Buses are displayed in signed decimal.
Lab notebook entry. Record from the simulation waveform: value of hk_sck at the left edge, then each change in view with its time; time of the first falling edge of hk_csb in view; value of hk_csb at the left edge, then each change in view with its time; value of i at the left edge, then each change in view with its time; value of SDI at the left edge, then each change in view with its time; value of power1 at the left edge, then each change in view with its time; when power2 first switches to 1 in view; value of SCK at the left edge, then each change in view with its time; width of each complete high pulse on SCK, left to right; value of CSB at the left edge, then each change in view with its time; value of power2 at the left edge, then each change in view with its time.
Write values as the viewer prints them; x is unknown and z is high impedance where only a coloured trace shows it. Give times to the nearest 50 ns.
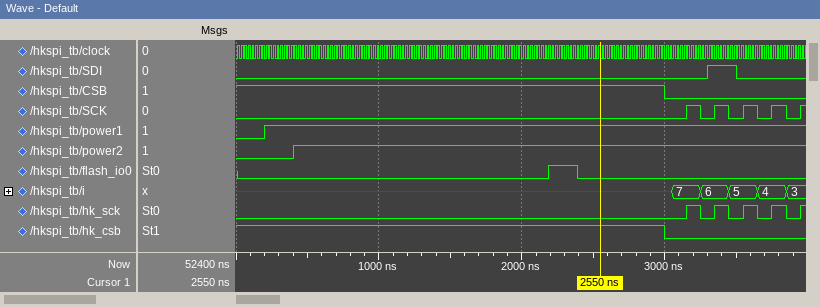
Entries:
0, 1 at 3150 ns, 0 at 3250 ns, 1 at 3350 ns, 0 at 3450 ns, 1 at 3550 ns, 0 at 3650 ns, 1 at 3750 ns, 0 at 3850 ns, 1 at 3950 ns
3000 ns
1, 0 at 3000 ns
x, 7 at 3050 ns, 6 at 3250 ns, 5 at 3450 ns, 4 at 3650 ns, 3 at 3850 ns
0, 1 at 3300 ns, 0 at 3500 ns
0, 1 at 200 ns
400 ns
0, 1 at 3150 ns, 0 at 3250 ns, 1 at 3350 ns, 0 at 3450 ns, 1 at 3550 ns, 0 at 3650 ns, 1 at 3750 ns, 0 at 3850 ns, 1 at 3950 ns
100 ns, 100 ns, 100 ns, 100 ns
1, 0 at 3000 ns
0, 1 at 400 ns
